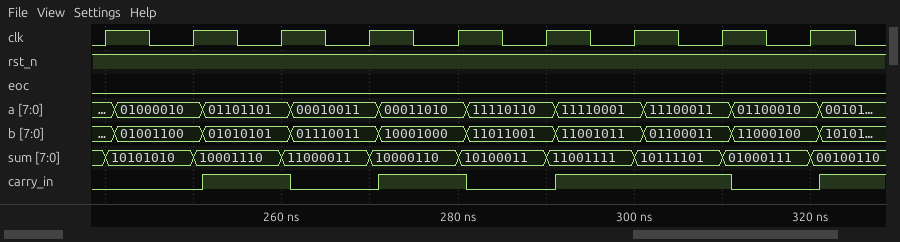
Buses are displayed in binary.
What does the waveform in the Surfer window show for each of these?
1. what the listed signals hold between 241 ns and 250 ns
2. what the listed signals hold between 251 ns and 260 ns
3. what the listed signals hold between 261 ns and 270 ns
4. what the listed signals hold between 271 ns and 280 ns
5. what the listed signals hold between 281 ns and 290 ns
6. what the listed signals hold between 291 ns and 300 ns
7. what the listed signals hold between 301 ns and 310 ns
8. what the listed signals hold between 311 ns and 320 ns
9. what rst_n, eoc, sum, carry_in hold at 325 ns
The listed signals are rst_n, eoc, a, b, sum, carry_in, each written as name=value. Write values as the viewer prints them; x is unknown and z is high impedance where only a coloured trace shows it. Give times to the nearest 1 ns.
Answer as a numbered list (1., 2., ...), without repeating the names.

1. rst_n=1, eoc=0, a=01000010, b=01001100, sum=10101010, carry_in=0
2. rst_n=1, eoc=0, a=01101101, b=01010101, sum=10001110, carry_in=1
3. rst_n=1, eoc=0, a=00010011, b=01110011, sum=11000011, carry_in=0
4. rst_n=1, eoc=0, a=00011010, b=10001000, sum=10000110, carry_in=1
5. rst_n=1, eoc=0, a=11110110, b=11011001, sum=10100011, carry_in=0
6. rst_n=1, eoc=0, a=11110001, b=11001011, sum=11001111, carry_in=1
7. rst_n=1, eoc=0, a=11100011, b=01100011, sum=10111101, carry_in=1
8. rst_n=1, eoc=0, a=01100010, b=11000100, sum=01000111, carry_in=0
9. rst_n=1, eoc=0, sum=00100110, carry_in=1
